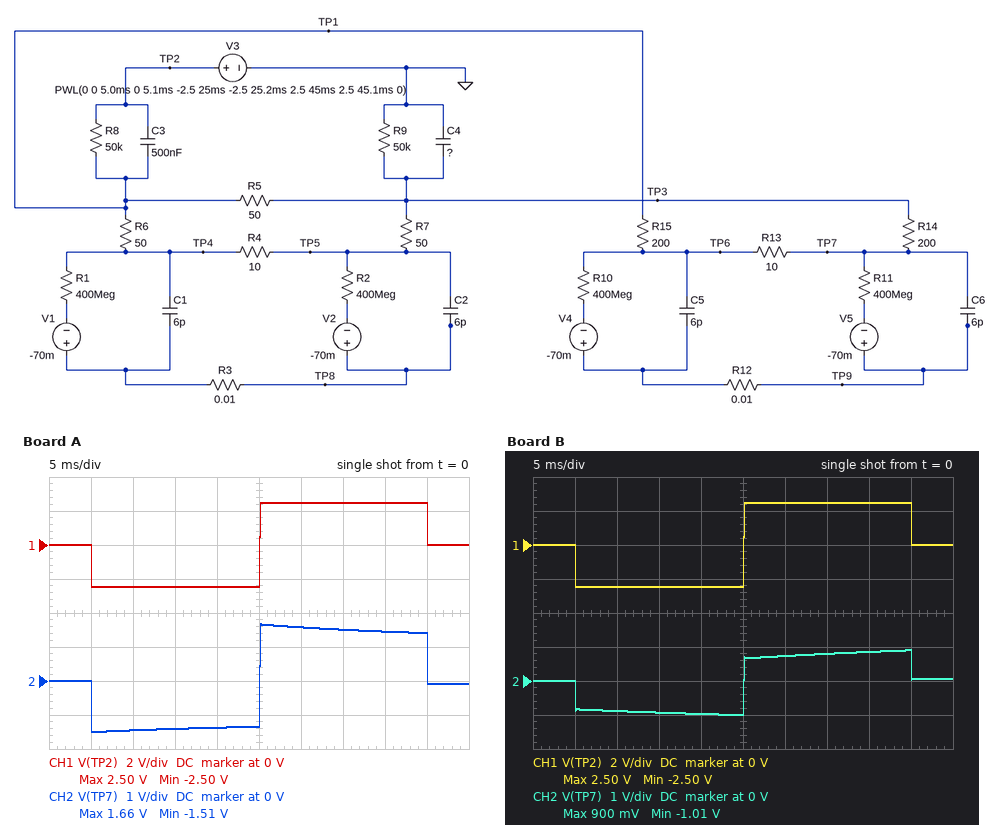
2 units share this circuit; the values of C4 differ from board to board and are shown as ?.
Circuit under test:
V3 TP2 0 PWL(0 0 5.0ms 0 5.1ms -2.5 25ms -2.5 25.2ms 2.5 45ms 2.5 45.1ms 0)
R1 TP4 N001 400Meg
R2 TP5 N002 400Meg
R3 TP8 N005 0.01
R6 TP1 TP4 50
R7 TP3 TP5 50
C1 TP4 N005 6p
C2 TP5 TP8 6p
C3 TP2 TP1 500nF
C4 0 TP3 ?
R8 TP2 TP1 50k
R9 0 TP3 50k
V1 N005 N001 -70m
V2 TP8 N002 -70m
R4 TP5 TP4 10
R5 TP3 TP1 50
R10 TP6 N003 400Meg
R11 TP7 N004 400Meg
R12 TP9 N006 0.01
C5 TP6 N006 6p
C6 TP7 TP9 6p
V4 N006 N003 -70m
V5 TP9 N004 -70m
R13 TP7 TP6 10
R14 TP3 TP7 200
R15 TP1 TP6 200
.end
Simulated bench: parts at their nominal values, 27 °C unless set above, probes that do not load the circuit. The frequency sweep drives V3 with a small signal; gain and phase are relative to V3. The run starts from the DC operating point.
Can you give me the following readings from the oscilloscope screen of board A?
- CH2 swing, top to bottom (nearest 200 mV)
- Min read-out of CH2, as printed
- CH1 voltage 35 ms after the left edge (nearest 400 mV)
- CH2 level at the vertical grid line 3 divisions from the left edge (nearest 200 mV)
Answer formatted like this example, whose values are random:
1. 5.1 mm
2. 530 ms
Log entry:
1. 3.2 V
2. -1.51 V
3. 2.4 V
4. -1.4 V
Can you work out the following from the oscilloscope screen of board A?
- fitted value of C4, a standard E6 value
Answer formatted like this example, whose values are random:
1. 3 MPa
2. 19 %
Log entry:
1. 330 nF
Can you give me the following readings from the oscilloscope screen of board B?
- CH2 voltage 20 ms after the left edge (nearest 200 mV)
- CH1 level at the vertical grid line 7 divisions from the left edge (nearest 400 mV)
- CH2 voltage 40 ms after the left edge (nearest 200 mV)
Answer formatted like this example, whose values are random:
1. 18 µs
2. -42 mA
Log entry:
1. -1.0 V
2. 2.4 V
3. 800 mV
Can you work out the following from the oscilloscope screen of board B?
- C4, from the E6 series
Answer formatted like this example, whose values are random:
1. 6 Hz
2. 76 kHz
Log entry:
1. 1 µF
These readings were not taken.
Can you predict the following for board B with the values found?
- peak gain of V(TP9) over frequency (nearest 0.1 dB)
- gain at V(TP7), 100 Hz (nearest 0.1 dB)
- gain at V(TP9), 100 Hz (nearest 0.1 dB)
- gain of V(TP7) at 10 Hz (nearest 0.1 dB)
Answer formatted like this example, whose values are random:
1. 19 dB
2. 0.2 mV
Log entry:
1. -6.0 dB
2. -9.5 dB
3. -9.5 dB
4. -8.8 dB
